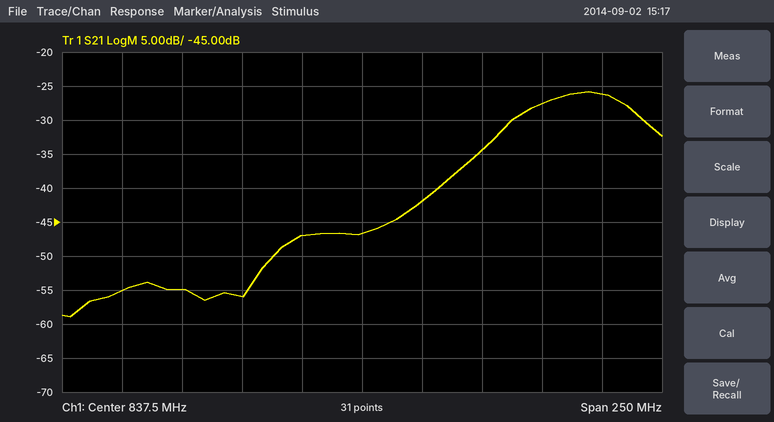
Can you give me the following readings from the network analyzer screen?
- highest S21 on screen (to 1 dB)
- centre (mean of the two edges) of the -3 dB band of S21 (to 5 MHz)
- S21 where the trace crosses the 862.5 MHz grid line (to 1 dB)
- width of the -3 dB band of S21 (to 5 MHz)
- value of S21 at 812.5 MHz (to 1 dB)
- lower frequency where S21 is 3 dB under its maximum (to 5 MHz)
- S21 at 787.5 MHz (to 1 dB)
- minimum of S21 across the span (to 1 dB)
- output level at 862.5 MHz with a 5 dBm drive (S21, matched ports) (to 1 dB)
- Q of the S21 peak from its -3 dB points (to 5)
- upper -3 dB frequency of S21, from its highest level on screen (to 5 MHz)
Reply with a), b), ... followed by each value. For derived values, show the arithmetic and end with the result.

a) -26 dB
b) 930 MHz
c) -42 dB
d) 950 MHz − 905 MHz = 45 MHz
e) -47 dB
f) 905 MHz
g) -56 dB
h) -59 dB
i) 5 dBm + (-42 dB) = -37 dBm
j) 927.5 MHz / 45 MHz ≈ 20.6, so 20 to the nearest 5
k) 950 MHz
